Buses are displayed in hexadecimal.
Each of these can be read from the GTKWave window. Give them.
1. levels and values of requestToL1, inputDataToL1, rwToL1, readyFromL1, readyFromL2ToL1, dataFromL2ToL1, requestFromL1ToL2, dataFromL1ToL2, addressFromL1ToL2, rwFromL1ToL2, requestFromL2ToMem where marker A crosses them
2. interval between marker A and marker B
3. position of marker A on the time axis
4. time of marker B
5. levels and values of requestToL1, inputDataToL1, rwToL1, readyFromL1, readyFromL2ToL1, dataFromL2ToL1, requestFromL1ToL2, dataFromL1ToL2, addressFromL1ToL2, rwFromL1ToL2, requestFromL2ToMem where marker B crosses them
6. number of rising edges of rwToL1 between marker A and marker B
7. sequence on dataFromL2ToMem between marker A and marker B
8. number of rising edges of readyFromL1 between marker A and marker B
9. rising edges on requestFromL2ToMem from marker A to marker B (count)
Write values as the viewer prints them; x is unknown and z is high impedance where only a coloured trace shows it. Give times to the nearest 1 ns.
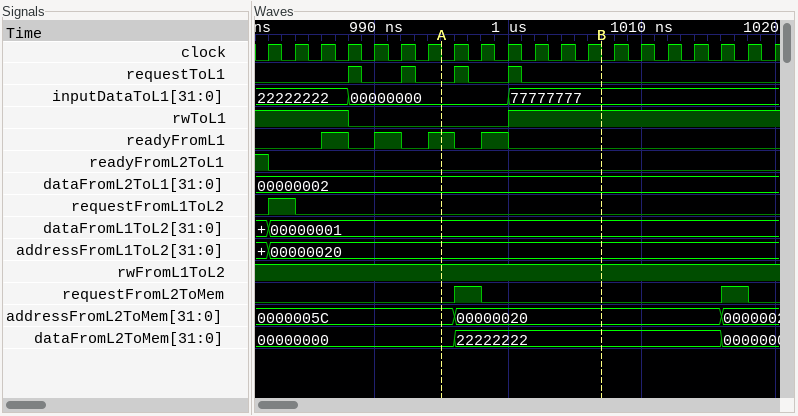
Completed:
requestToL1=0, inputDataToL1=00000000, rwToL1=0, readyFromL1=1, readyFromL2ToL1=0, dataFromL2ToL1=00000002, requestFromL1ToL2=0, dataFromL1ToL2=00000001, addressFromL1ToL2=00000020, rwFromL1ToL2=1, requestFromL2ToMem=0
12 ns
995 ns
1007 ns
requestToL1=0, inputDataToL1=77777777, rwToL1=1, readyFromL1=0, readyFromL2ToL1=0, dataFromL2ToL1=00000002, requestFromL1ToL2=0, dataFromL1ToL2=00000001, addressFromL1ToL2=00000020, rwFromL1ToL2=1, requestFromL2ToMem=0
1
00000000, 22222222
1
1
